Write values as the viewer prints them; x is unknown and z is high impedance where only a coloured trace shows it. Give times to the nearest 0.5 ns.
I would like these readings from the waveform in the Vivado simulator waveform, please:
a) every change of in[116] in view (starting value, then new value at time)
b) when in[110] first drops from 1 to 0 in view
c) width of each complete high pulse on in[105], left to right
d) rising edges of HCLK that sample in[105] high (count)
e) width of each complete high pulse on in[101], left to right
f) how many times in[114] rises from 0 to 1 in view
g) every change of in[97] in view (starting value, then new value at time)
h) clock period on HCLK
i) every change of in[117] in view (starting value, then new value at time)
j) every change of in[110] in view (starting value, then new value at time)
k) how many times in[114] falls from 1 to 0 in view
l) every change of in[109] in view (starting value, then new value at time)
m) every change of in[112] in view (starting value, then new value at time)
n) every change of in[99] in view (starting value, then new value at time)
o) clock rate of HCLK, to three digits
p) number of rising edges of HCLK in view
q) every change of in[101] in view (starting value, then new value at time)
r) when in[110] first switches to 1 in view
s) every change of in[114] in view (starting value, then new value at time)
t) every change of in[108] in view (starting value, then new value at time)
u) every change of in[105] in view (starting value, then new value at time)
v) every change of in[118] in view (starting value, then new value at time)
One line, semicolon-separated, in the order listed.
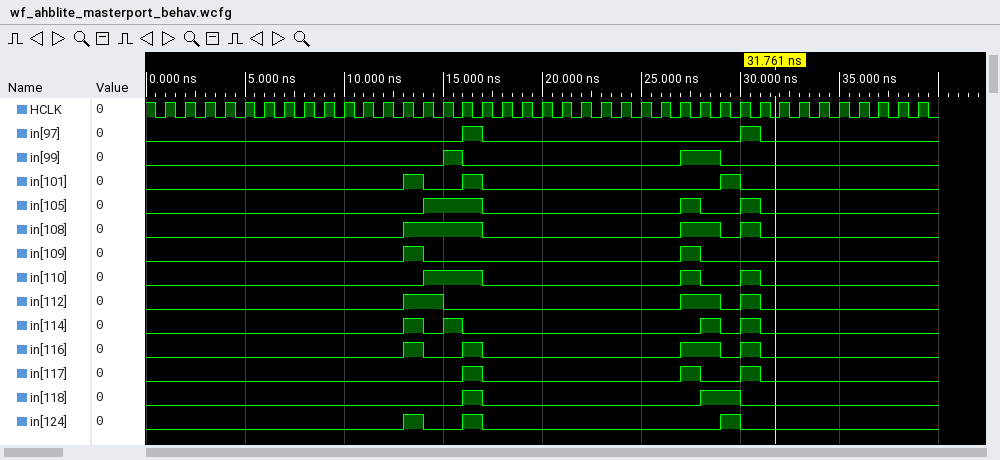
0, 1 at 13 ns, 0 at 14 ns, 1 at 16 ns, 0 at 17 ns, 1 at 27 ns, 0 at 29 ns, 1 at 30 ns, 0 at 31 ns; 17 ns; 3 ns, 1 ns, 1 ns; 5; 1 ns, 1 ns, 1 ns; 4; 0, 1 at 16 ns, 0 at 17 ns, 1 at 30 ns, 0 at 31 ns; 1 ns; 0, 1 at 16 ns, 0 at 17 ns, 1 at 27 ns, 0 at 28 ns, 1 at 30 ns, 0 at 31 ns; 0, 1 at 14 ns, 0 at 17 ns, 1 at 27 ns, 0 at 28 ns, 1 at 30 ns, 0 at 31 ns; 4; 0, 1 at 13 ns, 0 at 14 ns, 1 at 27 ns, 0 at 28 ns; 0, 1 at 13 ns, 0 at 15 ns, 1 at 27 ns, 0 at 29 ns, 1 at 30 ns, 0 at 31 ns; 0, 1 at 15 ns, 0 at 16 ns, 1 at 27 ns, 0 at 29 ns; 1.00 GHz; 39; 0, 1 at 13 ns, 0 at 14 ns, 1 at 16 ns, 0 at 17 ns, 1 at 29 ns, 0 at 30 ns; 14 ns; 0, 1 at 13 ns, 0 at 14 ns, 1 at 15 ns, 0 at 16 ns, 1 at 28 ns, 0 at 29 ns, 1 at 30 ns, 0 at 31 ns; 0, 1 at 13 ns, 0 at 17 ns, 1 at 27 ns, 0 at 29 ns, 1 at 30 ns, 0 at 31 ns; 0, 1 at 14 ns, 0 at 17 ns, 1 at 27 ns, 0 at 28 ns, 1 at 30 ns, 0 at 31 ns; 0, 1 at 16 ns, 0 at 17 ns, 1 at 28 ns, 0 at 30 ns
